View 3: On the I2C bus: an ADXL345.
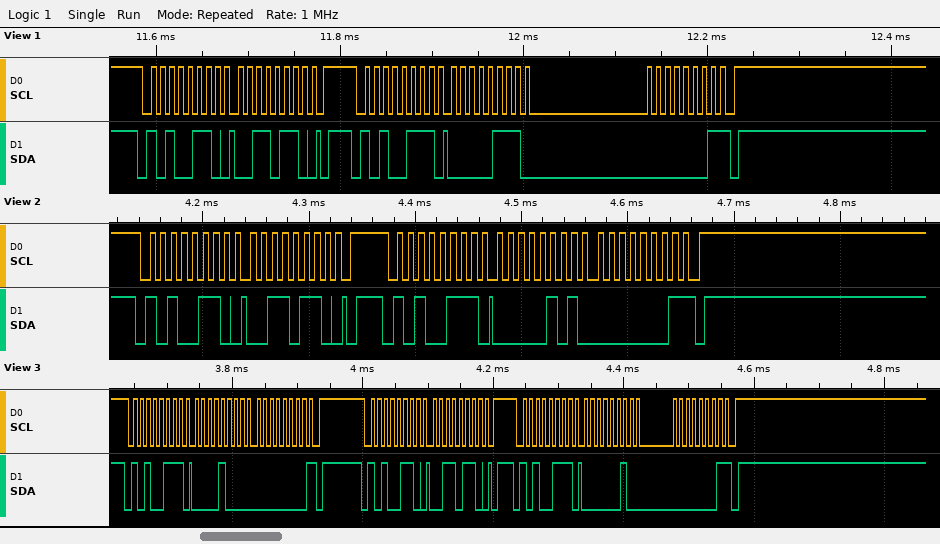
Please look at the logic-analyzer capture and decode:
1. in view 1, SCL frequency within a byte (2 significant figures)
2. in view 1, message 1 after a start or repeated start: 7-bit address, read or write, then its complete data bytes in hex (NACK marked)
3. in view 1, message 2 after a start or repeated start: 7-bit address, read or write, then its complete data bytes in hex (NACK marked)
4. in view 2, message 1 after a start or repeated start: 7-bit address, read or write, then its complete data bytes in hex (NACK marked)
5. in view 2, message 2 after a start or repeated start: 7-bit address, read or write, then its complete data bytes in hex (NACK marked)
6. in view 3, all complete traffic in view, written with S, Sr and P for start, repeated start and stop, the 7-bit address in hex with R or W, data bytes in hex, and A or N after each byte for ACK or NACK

100 kHz
0x53 write: 36
0x53 read: 07 01 NACK
0x53 write: 36
0x53 read: 05 01 NACK
S 53R A 08 A 00 N P S 53W A 36 A P S 53R A 02 A 01 N P
